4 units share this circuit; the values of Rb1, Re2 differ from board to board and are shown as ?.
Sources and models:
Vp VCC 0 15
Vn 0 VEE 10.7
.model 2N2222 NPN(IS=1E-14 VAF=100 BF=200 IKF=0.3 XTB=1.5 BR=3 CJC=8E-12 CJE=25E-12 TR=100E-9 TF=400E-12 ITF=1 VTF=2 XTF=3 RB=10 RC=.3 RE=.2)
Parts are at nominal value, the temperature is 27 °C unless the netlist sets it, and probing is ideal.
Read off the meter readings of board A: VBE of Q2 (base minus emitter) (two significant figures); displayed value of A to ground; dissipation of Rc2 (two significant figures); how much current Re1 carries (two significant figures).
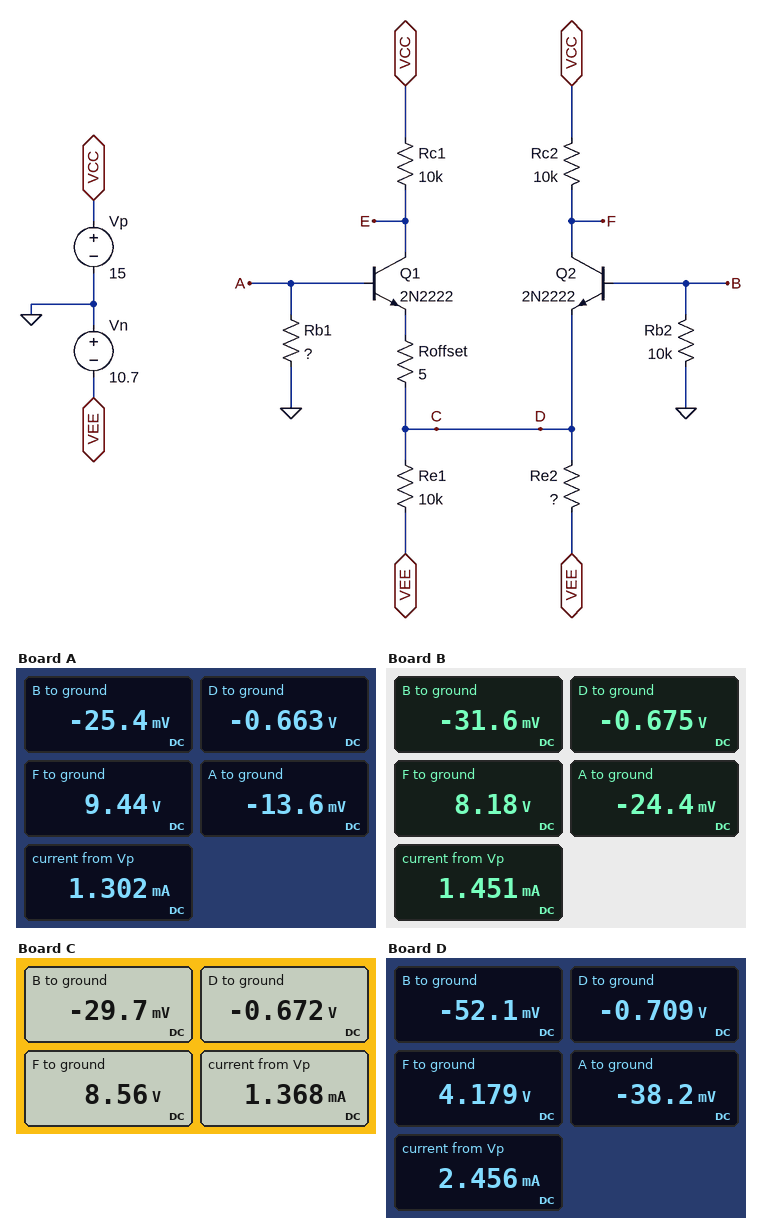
640 mV
-13.6 mV
3.1 mW
1.0 mA
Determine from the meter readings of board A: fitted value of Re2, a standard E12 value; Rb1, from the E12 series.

33 kΩ
3.9 kΩ
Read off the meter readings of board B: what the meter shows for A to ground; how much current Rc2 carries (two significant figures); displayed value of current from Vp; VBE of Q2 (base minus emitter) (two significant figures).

-24.4 mV
680 µA
1.451 mA
640 mV
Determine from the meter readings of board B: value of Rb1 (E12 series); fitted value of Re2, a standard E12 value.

6.8 kΩ
22 kΩ
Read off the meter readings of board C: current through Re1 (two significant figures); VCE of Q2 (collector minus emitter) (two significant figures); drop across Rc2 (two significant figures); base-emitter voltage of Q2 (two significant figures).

1.0 mA
9.2 V
6.4 V
640 mV
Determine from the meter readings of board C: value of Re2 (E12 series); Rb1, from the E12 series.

27 kΩ
6.8 kΩ
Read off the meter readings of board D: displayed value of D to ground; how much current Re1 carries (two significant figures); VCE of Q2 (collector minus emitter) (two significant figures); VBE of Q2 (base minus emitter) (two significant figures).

-0.709 V
1.0 mA
4.9 V
660 mV
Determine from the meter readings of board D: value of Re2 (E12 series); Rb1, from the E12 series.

6.8 kΩ
5.6 kΩ
